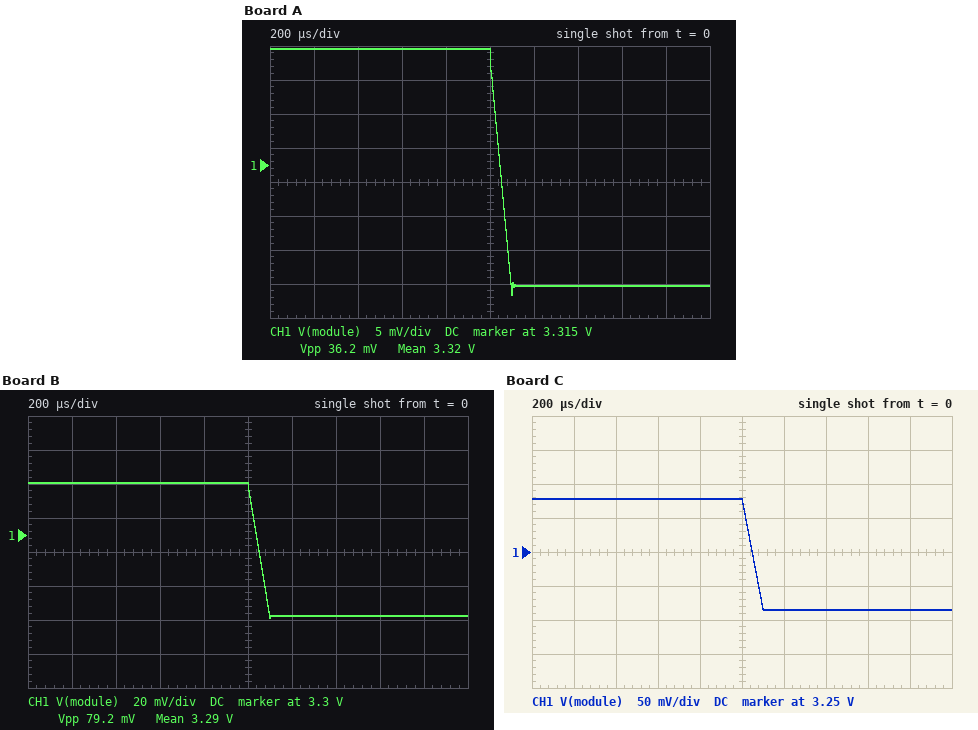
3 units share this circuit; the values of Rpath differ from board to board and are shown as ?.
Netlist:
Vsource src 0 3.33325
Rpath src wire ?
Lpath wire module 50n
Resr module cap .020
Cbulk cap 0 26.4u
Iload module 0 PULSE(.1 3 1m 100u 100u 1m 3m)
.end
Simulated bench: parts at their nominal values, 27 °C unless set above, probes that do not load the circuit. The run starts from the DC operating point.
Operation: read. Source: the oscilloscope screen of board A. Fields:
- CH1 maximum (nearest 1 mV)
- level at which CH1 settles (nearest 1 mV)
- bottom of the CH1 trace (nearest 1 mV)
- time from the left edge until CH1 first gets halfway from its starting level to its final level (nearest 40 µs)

3.332 V
3.297 V
3.296 V
1.04 ms
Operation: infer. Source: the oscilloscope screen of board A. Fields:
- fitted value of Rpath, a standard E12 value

0.012 Ω
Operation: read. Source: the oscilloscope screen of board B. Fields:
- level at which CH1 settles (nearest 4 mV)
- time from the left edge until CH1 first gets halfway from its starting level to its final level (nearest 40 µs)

3.252 V
1.04 ms
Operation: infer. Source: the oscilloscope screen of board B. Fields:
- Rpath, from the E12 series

0.027 Ω
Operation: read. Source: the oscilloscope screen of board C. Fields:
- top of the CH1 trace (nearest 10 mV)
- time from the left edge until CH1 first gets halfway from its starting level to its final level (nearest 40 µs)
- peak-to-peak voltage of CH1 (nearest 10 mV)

3.33 V
1.04 ms
160 mV
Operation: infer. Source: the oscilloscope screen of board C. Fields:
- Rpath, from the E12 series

0.056 Ω
